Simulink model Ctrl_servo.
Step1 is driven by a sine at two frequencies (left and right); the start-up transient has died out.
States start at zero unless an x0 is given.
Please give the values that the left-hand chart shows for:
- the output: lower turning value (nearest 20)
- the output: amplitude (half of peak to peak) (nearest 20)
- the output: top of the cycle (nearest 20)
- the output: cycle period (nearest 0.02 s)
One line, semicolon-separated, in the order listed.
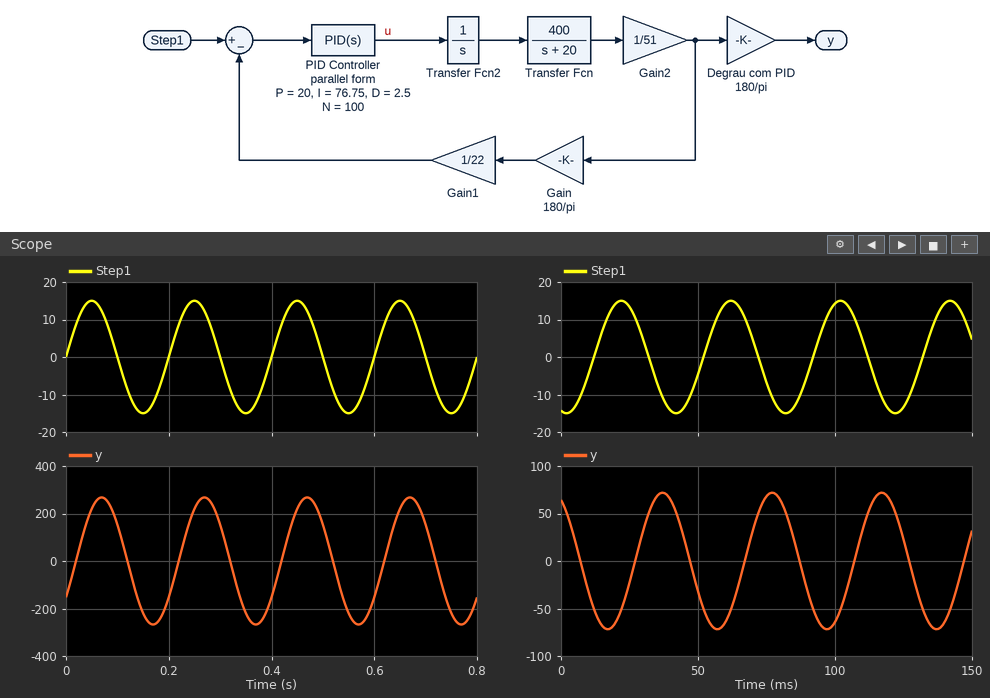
-260; 260; 260; 0.20 s
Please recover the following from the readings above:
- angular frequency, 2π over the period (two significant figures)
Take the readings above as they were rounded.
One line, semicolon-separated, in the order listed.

31 rad/s
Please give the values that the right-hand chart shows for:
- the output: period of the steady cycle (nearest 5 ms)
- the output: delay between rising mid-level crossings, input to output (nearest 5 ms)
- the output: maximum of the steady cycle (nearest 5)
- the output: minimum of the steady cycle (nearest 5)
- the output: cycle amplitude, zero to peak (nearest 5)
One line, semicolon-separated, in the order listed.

40 ms; 15 ms; 70; -70; 70
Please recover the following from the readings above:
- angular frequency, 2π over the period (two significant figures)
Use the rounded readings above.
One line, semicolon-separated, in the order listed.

0.16 rad/ms
